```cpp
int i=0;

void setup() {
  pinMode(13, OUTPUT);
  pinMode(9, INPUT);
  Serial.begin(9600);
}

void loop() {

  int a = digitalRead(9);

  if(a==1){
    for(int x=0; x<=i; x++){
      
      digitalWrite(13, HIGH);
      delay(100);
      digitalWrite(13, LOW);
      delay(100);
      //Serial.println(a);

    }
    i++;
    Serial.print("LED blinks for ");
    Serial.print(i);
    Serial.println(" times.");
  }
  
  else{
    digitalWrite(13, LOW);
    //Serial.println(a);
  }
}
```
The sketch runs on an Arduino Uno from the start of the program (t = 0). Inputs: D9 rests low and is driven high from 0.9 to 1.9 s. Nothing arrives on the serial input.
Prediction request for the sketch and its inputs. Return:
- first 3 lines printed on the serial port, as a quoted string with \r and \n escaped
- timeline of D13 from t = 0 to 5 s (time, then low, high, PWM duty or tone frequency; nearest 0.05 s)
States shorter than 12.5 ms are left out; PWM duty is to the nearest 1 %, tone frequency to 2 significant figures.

"LED blinks for 1 times.\r\nLED blinks for 2 times.\r\nLED blinks for 3 times.\r\n"
0 s low; 0.9 s high; 1 s low; 1.1 s high; 1.2 s low; 1.3 s high; 1.4 s low; 1.5 s high; 1.6 s low; 1.7 s high; 1.8 s low; 1.9 s high; 2 s low
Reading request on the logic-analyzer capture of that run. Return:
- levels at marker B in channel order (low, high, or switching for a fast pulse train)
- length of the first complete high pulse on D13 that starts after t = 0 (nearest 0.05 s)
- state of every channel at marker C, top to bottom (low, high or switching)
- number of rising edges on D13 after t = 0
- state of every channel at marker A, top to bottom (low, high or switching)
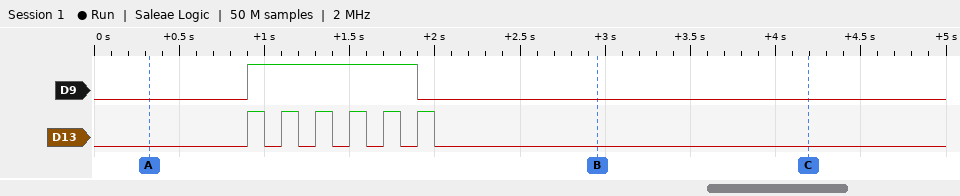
D9 low, D13 low
0.10 s
D9 low, D13 low
6
D9 low, D13 low
